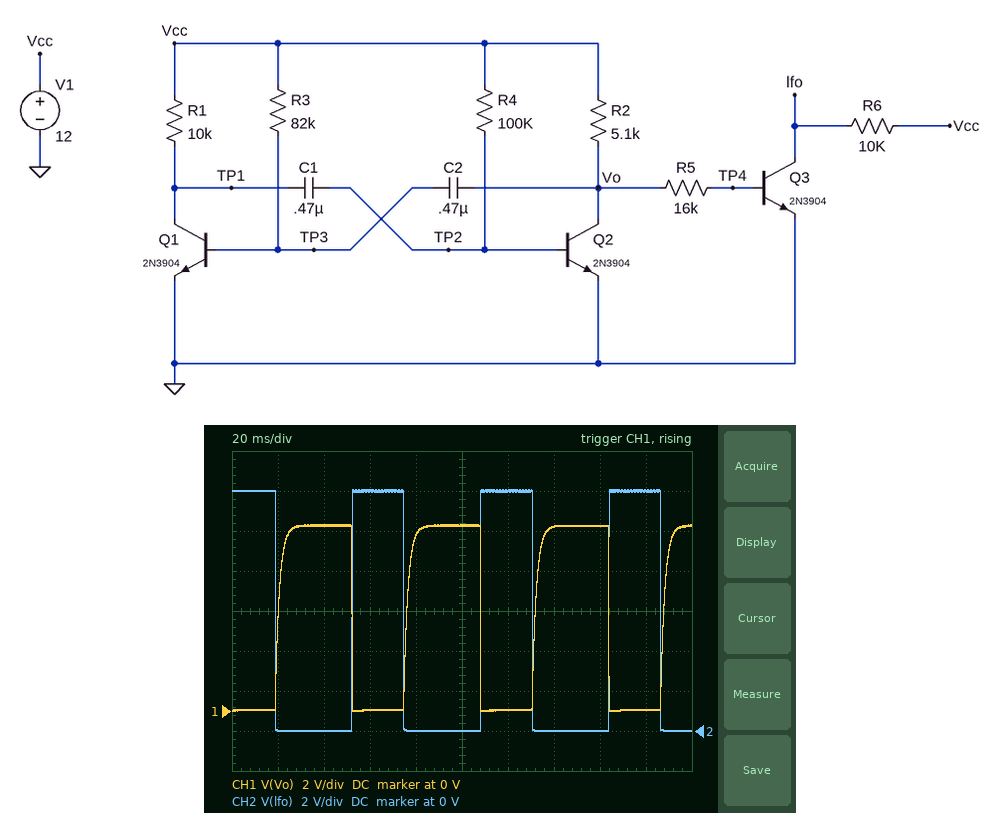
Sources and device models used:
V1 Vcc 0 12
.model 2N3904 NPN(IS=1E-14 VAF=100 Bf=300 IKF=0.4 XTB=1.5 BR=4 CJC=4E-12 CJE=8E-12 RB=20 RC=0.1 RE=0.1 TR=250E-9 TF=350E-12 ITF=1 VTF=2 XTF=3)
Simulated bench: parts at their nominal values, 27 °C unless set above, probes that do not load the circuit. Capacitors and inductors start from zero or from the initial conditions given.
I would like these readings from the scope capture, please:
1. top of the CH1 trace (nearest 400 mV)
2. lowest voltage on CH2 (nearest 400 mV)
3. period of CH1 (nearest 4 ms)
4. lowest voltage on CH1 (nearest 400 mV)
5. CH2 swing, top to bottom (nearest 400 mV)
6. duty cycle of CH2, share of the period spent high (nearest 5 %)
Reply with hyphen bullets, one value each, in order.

- 9.2 V
- 0 V
- 56 ms
- 0 V
- 12.0 V
- 40 %
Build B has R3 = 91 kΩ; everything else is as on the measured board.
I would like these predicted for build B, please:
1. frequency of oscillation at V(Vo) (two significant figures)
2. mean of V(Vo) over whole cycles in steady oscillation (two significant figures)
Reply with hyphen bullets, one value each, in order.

- 17 Hz
- 5.0 V
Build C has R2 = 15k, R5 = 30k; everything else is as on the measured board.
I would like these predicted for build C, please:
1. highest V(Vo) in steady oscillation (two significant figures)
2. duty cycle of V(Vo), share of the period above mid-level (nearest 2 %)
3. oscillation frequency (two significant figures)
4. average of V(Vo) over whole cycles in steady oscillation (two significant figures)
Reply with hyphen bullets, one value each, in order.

- 8.2 V
- 56 %
- 19 Hz
- 4.4 V
